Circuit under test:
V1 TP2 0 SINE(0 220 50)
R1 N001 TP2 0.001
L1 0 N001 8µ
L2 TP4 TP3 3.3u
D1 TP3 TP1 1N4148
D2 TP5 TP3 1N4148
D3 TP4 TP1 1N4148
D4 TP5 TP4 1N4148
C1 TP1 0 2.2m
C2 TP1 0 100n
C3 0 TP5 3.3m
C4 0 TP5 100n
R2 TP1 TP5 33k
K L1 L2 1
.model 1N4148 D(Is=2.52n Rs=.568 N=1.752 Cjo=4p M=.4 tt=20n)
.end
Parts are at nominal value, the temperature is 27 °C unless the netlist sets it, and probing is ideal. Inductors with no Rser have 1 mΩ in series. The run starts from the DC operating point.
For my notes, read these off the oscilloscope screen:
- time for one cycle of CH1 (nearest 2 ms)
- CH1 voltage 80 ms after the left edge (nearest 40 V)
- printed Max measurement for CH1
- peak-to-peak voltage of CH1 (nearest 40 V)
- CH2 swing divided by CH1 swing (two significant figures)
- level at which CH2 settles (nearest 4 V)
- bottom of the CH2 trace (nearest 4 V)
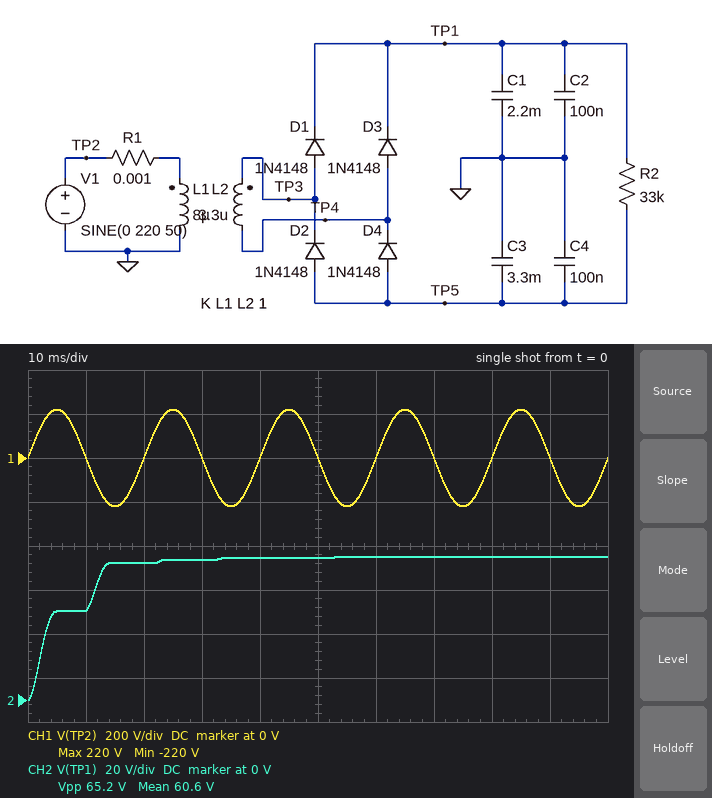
20 ms
0 V
220 V
440 V
0.15
64 V
0 V
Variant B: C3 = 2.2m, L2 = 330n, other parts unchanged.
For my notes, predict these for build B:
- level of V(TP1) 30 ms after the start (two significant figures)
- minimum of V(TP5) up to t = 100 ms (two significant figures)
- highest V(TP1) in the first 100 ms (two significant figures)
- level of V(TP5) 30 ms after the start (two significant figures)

16 V
-17 V
17 V
-16 V
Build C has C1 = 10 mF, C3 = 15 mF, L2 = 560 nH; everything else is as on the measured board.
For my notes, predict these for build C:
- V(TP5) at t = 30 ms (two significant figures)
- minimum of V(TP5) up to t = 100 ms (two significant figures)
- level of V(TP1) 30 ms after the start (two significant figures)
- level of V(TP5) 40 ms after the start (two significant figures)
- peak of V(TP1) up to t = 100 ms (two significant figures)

-14 V
-17 V
20 V
-15 V
25 V
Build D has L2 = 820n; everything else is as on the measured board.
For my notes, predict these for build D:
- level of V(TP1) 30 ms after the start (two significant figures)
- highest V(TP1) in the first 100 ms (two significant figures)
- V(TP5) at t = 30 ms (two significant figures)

31 V
32 V
-21 V
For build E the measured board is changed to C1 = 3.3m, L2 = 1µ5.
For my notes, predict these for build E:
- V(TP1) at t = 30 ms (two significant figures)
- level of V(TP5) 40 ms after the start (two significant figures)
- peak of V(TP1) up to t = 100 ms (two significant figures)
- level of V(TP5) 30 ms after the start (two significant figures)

35 V
-36 V
36 V
-35 V
